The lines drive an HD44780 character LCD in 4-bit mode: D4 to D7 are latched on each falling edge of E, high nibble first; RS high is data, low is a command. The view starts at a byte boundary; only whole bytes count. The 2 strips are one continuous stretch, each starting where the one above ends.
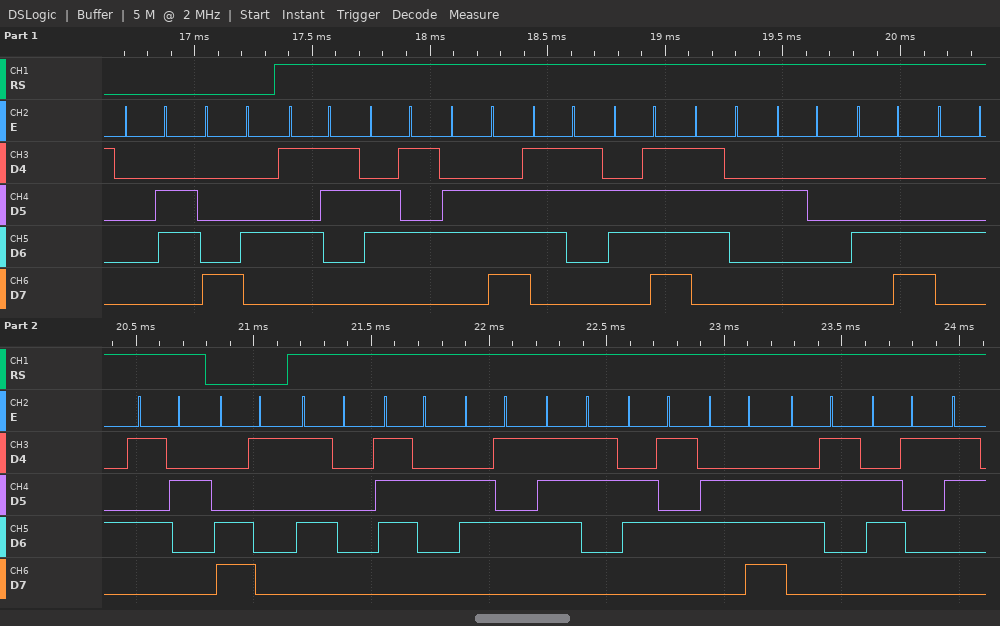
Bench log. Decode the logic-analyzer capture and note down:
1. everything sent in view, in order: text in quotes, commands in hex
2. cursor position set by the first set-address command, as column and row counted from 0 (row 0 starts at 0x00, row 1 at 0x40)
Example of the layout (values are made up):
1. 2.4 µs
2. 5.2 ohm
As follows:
1. 0x06 0x84 "Sensor LDR" 0xC1 "Presenca"
2. column 4, row 0
